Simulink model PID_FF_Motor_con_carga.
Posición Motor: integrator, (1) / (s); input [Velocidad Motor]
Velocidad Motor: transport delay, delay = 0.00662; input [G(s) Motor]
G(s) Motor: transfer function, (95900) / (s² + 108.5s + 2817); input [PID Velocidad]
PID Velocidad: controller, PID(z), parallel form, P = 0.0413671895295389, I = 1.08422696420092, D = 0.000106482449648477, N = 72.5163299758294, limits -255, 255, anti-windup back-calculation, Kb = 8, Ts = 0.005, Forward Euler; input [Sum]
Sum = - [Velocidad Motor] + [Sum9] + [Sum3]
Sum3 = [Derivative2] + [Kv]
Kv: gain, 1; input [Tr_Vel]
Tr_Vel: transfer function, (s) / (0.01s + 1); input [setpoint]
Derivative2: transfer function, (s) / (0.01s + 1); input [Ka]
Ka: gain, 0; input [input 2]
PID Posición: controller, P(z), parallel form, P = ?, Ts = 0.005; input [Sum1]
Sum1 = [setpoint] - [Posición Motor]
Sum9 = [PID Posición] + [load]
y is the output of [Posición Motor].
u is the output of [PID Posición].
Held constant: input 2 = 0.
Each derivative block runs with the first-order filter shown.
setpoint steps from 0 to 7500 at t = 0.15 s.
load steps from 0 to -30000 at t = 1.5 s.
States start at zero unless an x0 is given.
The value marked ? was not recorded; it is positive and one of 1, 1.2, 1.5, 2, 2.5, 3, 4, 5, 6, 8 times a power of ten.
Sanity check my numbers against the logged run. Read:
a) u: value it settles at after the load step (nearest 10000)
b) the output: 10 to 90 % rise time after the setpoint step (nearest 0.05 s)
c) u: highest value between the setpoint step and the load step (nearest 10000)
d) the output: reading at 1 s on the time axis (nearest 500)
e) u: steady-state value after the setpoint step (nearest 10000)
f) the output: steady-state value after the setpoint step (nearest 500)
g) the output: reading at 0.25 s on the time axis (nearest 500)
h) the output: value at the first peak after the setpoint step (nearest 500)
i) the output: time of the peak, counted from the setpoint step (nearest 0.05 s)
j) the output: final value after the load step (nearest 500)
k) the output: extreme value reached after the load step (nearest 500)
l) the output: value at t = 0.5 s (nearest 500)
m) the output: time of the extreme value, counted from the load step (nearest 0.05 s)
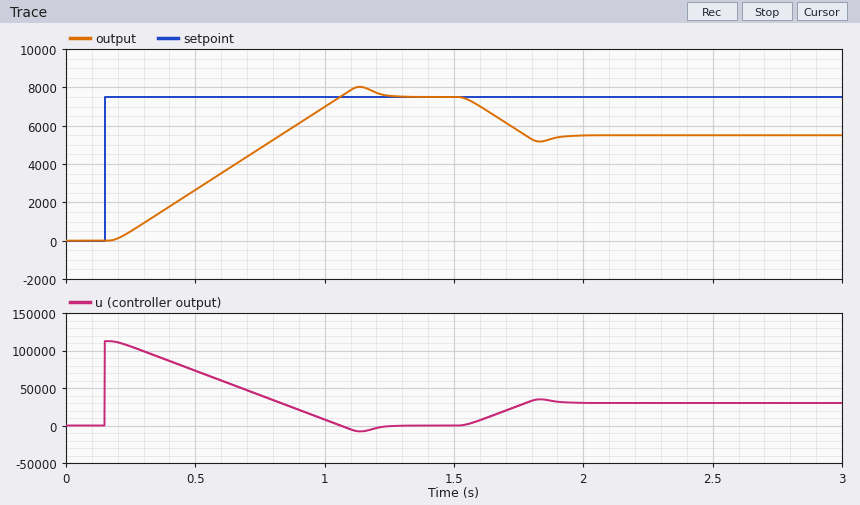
30000
0.70 s
110000
7000
0
7500
500
8000
1.00 s
5500
5000
2500
0.35 s
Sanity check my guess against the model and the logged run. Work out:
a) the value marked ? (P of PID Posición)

15
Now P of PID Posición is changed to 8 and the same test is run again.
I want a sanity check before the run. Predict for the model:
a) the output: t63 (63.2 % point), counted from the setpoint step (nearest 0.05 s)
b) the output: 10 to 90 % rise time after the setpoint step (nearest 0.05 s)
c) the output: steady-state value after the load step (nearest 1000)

0.60 s
0.70 s
4000
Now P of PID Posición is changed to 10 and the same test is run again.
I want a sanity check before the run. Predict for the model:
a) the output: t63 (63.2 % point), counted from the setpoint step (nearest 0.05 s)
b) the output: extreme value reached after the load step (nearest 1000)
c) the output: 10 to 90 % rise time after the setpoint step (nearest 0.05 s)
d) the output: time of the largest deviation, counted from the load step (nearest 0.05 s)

0.60 s
4000
0.70 s
0.45 s
